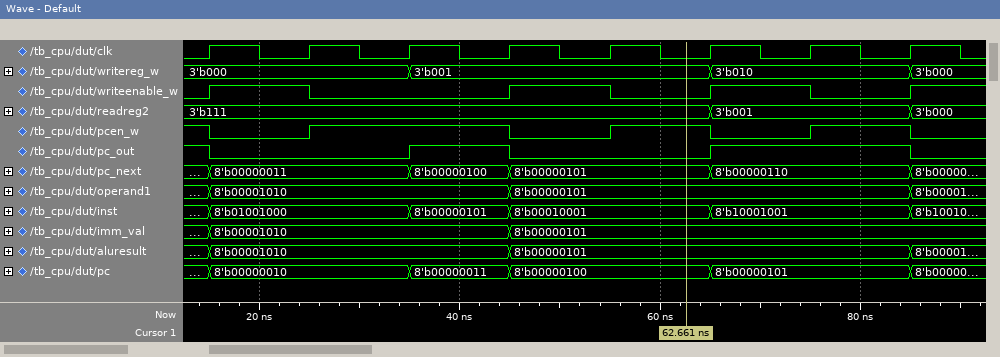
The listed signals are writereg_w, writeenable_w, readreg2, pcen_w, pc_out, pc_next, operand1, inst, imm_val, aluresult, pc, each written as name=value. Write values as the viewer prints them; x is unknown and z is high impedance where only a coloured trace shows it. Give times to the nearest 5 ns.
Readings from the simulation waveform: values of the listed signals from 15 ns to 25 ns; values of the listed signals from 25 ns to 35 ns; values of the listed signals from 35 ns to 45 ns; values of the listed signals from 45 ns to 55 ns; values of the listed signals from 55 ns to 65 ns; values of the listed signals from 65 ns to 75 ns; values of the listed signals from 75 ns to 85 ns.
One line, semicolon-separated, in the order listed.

writereg_w=3'b000, writeenable_w=1, readreg2=3'b111, pcen_w=0, pc_out=0, pc_next=8'b00000011, operand1=8'b00001010, inst=8'b01001000, imm_val=8'b00001010, aluresult=8'b00001010, pc=8'b00000010; writereg_w=3'b000, writeenable_w=0, readreg2=3'b111, pcen_w=1, pc_out=0, pc_next=8'b00000011, operand1=8'b00001010, inst=8'b01001000, imm_val=8'b00001010, aluresult=8'b00001010, pc=8'b00000010; writereg_w=3'b001, writeenable_w=0, readreg2=3'b111, pcen_w=1, pc_out=1, pc_next=8'b00000100, operand1=8'b00001010, inst=8'b00000101, imm_val=8'b00001010, aluresult=8'b00001010, pc=8'b00000011; writereg_w=3'b001, writeenable_w=1, readreg2=3'b111, pcen_w=0, pc_out=0, pc_next=8'b00000101, operand1=8'b00000101, inst=8'b00010001, imm_val=8'b00000101, aluresult=8'b00000101, pc=8'b00000100; writereg_w=3'b001, writeenable_w=0, readreg2=3'b111, pcen_w=1, pc_out=0, pc_next=8'b00000101, operand1=8'b00000101, inst=8'b00010001, imm_val=8'b00000101, aluresult=8'b00000101, pc=8'b00000100; writereg_w=3'b010, writeenable_w=1, readreg2=3'b001, pcen_w=0, pc_out=1, pc_next=8'b00000110, operand1=8'b00000101, inst=8'b10001001, imm_val=8'b00000101, aluresult=8'b00000101, pc=8'b00000101; writereg_w=3'b010, writeenable_w=0, readreg2=3'b001, pcen_w=1, pc_out=1, pc_next=8'b00000110, operand1=8'b00000101, inst=8'b10001001, imm_val=8'b00000101, aluresult=8'b00000101, pc=8'b00000101
